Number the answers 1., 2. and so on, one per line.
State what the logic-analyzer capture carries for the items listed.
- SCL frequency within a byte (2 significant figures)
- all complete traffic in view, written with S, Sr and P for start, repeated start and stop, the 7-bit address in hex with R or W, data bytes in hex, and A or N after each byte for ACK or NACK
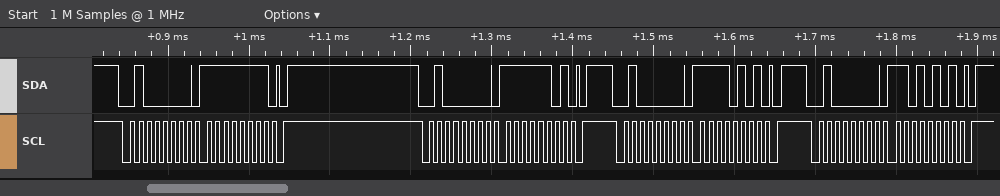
1. 100 kHz
2. S 20W A FF A P S 20W A FD A P S 20W A F5 A P S 20W A D5 A P
